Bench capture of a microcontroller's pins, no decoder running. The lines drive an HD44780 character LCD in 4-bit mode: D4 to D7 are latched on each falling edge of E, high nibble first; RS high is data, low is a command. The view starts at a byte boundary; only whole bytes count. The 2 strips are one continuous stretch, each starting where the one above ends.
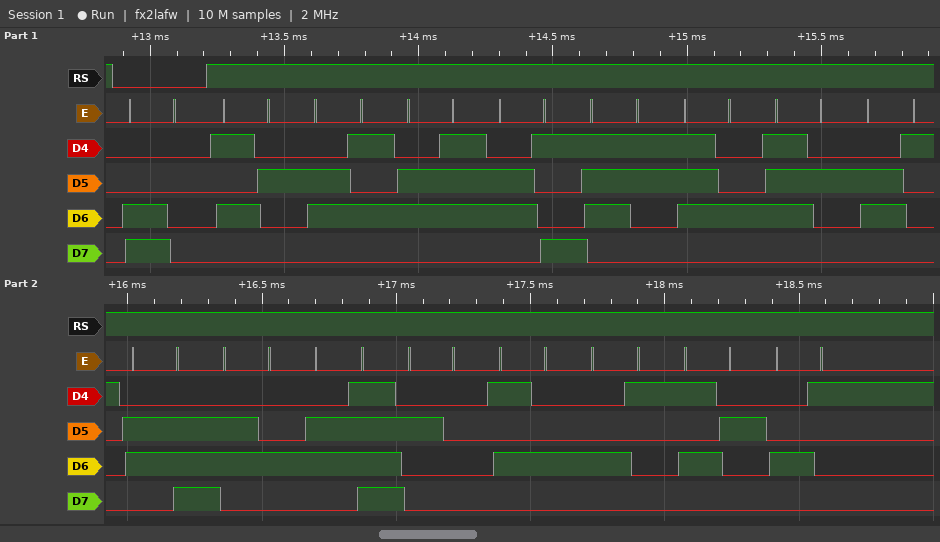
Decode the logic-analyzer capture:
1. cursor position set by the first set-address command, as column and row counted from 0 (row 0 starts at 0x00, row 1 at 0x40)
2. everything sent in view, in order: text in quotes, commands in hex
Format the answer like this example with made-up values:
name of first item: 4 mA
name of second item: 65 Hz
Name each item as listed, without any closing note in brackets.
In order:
cursor position set by the first set-address command, as column and row counted from 0: column 0, row 1
everything sent in view, in order: text in quotes, commands in hex: 0xC0 "Registrando TARA"
